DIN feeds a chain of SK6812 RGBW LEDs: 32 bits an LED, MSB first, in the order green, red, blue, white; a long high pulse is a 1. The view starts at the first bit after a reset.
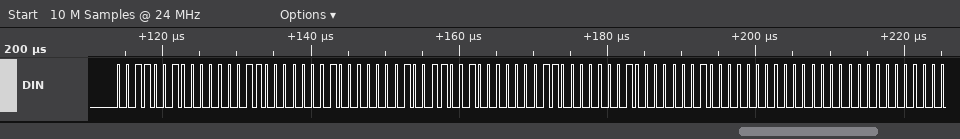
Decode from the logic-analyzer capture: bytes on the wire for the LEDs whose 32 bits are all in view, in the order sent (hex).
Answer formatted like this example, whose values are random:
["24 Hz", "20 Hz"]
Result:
["32 03 01 01 32 03 01 01"]
